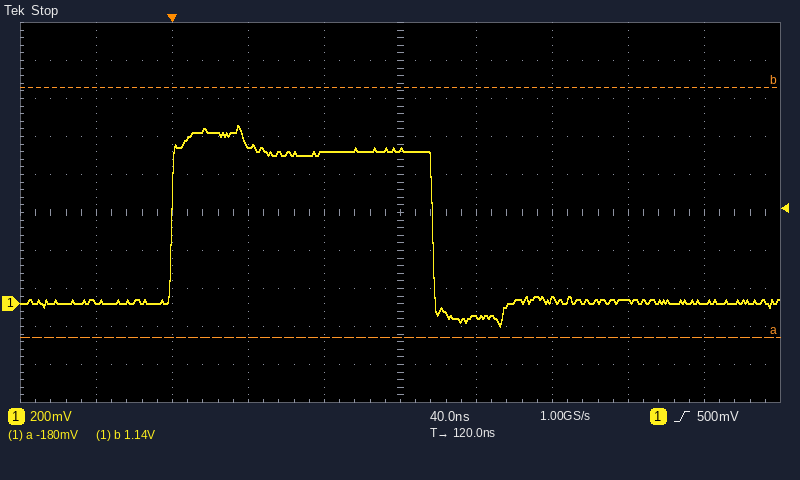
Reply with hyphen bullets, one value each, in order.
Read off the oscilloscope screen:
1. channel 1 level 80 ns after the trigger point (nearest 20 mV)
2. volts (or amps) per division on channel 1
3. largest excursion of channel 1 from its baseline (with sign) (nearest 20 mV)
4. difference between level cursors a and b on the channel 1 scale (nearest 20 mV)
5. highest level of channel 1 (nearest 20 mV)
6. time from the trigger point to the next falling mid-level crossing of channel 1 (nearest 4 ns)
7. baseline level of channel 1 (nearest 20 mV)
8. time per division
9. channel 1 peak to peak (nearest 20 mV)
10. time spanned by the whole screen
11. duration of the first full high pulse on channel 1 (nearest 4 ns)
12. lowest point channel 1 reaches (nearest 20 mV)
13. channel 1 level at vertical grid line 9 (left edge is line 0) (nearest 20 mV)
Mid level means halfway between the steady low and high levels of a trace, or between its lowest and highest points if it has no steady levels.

- 800 mV
- 200 mV
- +940 mV
- 1.32 V
- 940 mV
- 136 ns
- 0 mV
- 40 ns
- 1.06 V
- 400 ns
- 136 ns
- -120 mV
- 0 mV
